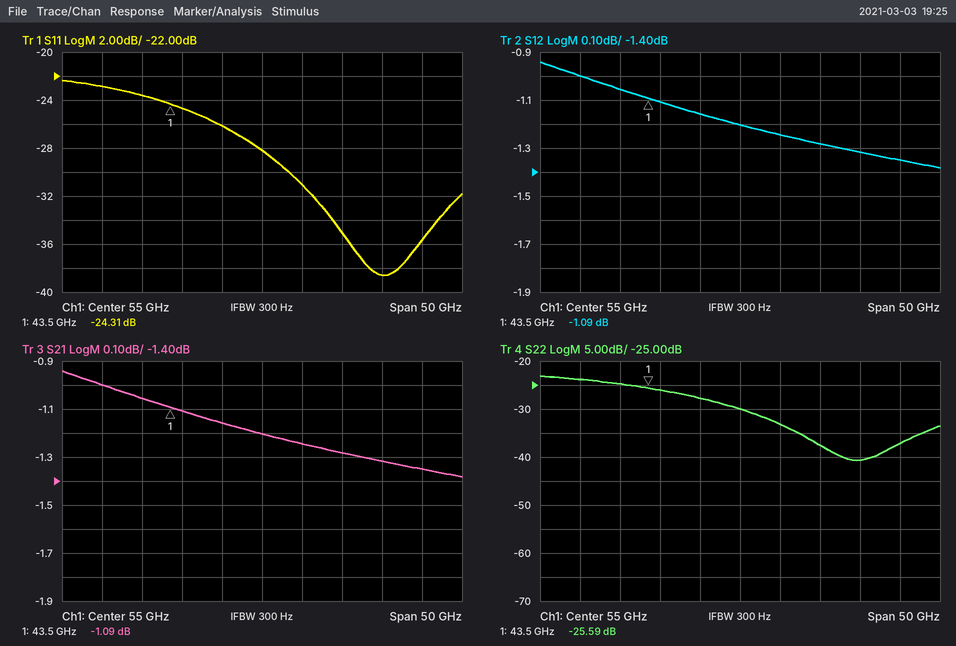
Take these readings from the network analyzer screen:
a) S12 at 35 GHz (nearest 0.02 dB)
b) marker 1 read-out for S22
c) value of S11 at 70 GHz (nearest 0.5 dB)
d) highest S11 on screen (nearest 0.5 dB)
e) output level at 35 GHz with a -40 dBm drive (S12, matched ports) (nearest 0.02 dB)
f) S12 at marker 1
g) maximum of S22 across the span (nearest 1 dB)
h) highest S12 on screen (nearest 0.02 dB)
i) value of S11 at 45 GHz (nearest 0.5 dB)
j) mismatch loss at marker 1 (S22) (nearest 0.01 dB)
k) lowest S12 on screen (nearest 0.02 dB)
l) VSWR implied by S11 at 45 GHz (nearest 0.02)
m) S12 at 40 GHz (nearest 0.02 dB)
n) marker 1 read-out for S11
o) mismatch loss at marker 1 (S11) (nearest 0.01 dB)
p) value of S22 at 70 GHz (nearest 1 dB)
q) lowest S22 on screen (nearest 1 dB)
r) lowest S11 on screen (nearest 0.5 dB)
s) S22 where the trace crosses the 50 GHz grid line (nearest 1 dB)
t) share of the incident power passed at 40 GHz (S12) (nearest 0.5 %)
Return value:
-1.00 dB
-25.59 dB
-38.5 dB
-22.5 dB
-41.00 dBm
-1.09 dB
-23 dB
-0.94 dB
-24.5 dB
0.01 dB
-1.38 dB
1.12
-1.06 dB
-24.31 dB
0.02 dB
-41 dB
-41 dB
-38.5 dB
-28 dB
78.5 %
